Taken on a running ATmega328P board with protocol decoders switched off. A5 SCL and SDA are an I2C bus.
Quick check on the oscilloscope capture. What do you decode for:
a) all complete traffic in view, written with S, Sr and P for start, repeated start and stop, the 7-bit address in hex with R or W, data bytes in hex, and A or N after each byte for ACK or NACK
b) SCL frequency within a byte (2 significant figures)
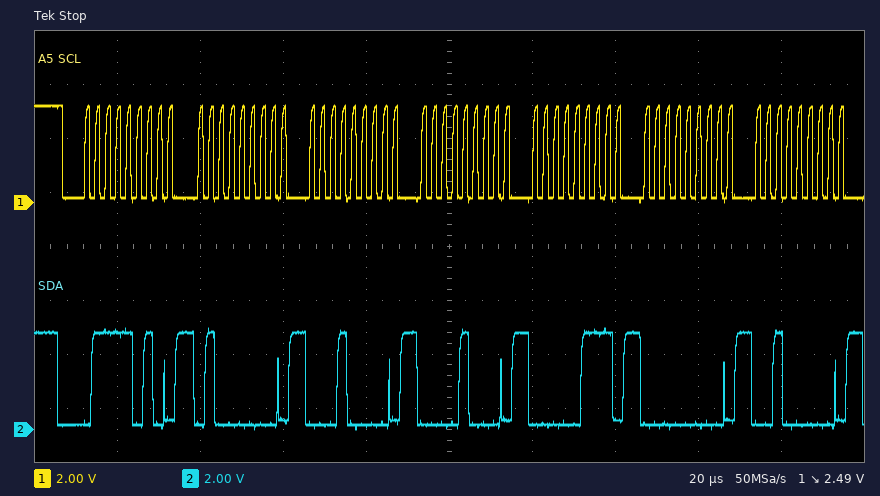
S 3DW A 40 A 10 A 08 A 07 A 00 A 20 A
400 kHz
